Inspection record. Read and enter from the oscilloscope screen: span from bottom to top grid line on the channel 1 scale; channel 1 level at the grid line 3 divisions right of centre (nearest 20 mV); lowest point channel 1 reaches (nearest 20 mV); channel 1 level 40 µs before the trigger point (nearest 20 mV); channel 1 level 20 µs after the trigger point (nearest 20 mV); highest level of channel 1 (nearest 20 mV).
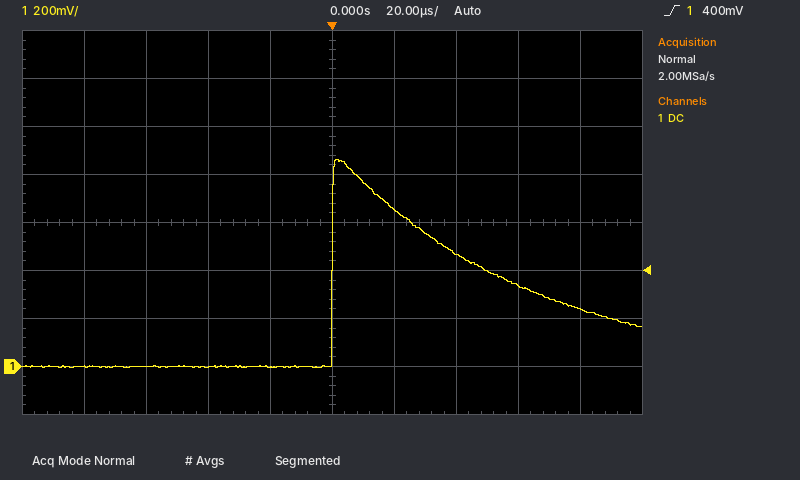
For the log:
1.6 V
340 mV
0 mV
0 mV
660 mV
860 mV
